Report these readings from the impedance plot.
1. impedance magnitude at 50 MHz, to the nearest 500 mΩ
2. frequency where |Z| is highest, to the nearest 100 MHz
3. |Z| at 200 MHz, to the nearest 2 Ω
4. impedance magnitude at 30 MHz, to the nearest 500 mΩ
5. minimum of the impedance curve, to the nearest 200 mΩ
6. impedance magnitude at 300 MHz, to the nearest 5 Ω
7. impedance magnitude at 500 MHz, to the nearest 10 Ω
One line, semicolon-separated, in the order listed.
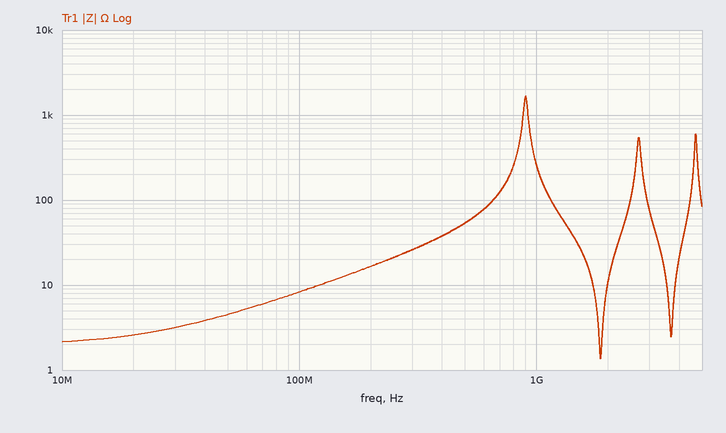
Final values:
4.5 Ω; 900 MHz; 16 Ω; 3.0 Ω; 1.4 Ω; 25 Ω; 50 Ω
